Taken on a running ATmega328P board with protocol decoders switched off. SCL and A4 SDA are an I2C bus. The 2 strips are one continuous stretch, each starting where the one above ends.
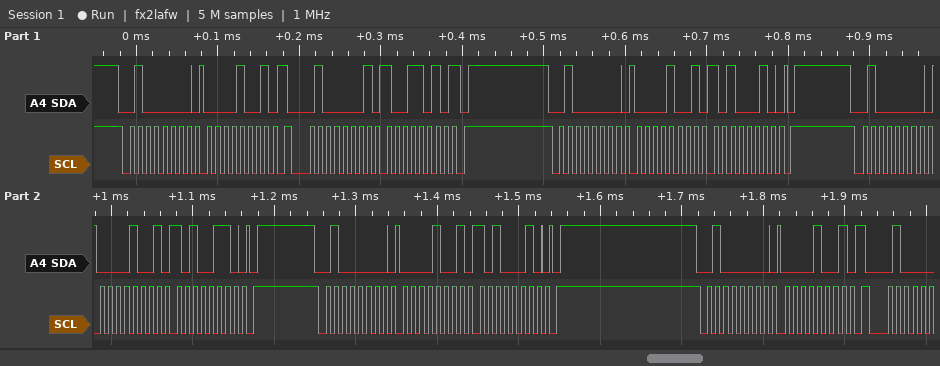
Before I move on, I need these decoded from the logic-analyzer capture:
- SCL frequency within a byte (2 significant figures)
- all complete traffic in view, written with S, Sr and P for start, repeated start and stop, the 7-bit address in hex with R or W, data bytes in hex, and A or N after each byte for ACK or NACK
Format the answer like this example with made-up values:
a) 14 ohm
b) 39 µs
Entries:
a) 100 kHz
b) S 20W A 09 A Sr 20R A 9A N P S 20W A 09 A A2 A P S 20W A 09 A A6 A P S 20W A 09 A A2 A P S 20W A 09 A
